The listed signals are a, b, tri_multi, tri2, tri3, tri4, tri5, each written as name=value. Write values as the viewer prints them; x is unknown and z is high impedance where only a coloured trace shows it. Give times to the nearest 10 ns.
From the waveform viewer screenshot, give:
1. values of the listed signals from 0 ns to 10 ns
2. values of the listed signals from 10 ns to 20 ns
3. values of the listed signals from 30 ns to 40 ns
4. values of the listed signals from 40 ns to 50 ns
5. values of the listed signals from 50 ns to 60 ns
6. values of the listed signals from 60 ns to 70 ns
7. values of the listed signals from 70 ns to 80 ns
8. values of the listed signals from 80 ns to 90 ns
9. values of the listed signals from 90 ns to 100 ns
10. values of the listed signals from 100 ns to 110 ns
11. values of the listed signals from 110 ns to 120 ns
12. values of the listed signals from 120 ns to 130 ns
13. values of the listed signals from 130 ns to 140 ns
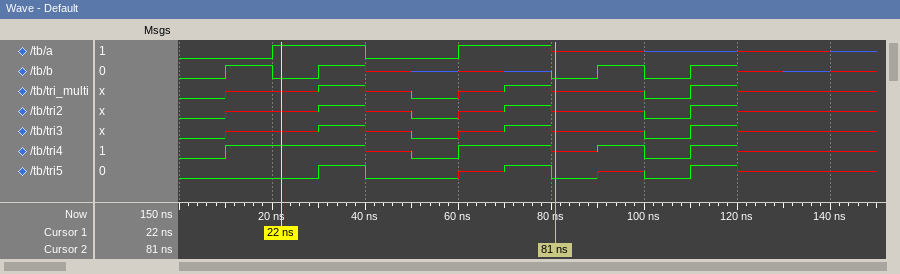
a=0, b=0, tri_multi=0, tri2=0, tri3=0, tri4=0, tri5=0
a=0, b=1, tri_multi=x, tri2=x, tri3=x, tri4=1, tri5=0
a=1, b=1, tri_multi=1, tri2=1, tri3=1, tri4=1, tri5=1
a=0, b=x, tri_multi=x, tri2=x, tri3=x, tri4=x, tri5=0
a=0, b=z, tri_multi=0, tri2=0, tri3=0, tri4=0, tri5=0
a=1, b=x, tri_multi=x, tri2=x, tri3=x, tri4=1, tri5=x
a=1, b=z, tri_multi=1, tri2=1, tri3=1, tri4=1, tri5=1
a=x, b=0, tri_multi=x, tri2=x, tri3=x, tri4=x, tri5=0
a=x, b=1, tri_multi=x, tri2=x, tri3=x, tri4=1, tri5=x
a=z, b=0, tri_multi=0, tri2=0, tri3=0, tri4=0, tri5=0
a=z, b=1, tri_multi=1, tri2=1, tri3=1, tri4=1, tri5=1
a=x, b=x, tri_multi=x, tri2=x, tri3=x, tri4=x, tri5=x
a=x, b=z, tri_multi=x, tri2=x, tri3=x, tri4=x, tri5=x
